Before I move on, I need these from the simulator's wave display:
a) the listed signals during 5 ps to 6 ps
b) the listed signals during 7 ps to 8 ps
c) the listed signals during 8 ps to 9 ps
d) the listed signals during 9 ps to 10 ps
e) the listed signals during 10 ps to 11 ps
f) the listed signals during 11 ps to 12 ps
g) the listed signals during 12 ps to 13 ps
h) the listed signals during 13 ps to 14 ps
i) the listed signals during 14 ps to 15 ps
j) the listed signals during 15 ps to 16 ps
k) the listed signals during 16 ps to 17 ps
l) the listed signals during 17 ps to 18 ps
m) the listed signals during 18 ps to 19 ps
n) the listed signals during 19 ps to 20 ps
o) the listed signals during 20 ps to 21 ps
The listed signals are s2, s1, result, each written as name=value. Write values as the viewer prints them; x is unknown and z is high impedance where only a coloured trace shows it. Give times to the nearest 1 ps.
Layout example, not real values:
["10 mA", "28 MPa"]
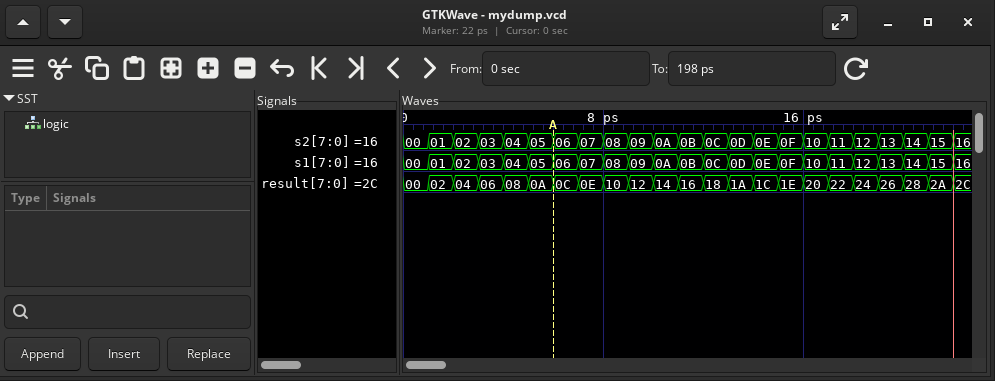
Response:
["s2=05, s1=05, result=0A", "s2=07, s1=07, result=0E", "s2=08, s1=08, result=10", "s2=09, s1=09, result=12", "s2=0A, s1=0A, result=14", "s2=0B, s1=0B, result=16", "s2=0C, s1=0C, result=18", "s2=0D, s1=0D, result=1A", "s2=0E, s1=0E, result=1C", "s2=0F, s1=0F, result=1E", "s2=10, s1=10, result=20", "s2=11, s1=11, result=22", "s2=12, s1=12, result=24", "s2=13, s1=13, result=26", "s2=14, s1=14, result=28"]
